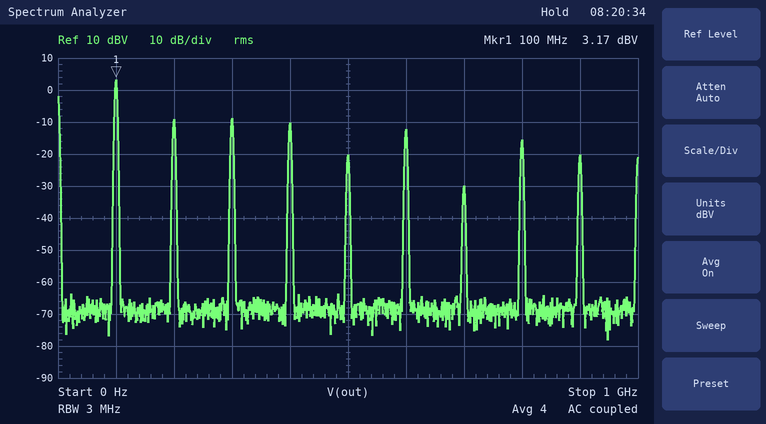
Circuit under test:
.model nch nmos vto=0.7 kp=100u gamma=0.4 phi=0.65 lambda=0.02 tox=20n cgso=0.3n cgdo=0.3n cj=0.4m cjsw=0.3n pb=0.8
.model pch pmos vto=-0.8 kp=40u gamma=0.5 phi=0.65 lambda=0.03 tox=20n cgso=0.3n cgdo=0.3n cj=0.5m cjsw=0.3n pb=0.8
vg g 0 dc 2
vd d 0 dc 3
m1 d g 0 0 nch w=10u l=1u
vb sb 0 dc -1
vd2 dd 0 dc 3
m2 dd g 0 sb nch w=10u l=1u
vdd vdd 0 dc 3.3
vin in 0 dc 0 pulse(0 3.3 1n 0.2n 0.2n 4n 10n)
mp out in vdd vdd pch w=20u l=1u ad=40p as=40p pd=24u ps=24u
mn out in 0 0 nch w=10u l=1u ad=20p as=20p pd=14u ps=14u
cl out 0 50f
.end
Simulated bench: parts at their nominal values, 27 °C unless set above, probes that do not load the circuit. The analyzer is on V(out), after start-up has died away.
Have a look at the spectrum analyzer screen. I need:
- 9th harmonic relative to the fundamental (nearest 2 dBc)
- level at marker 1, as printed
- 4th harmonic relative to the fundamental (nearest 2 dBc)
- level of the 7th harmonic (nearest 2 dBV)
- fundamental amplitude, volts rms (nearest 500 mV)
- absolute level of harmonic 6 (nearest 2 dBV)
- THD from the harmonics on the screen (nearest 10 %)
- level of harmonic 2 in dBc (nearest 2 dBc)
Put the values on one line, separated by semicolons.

-24 dBc; 3.17 dBV; -14 dBc; -30 dBV; 1.5 V; -12 dBV; 50 %; -12 dBc
